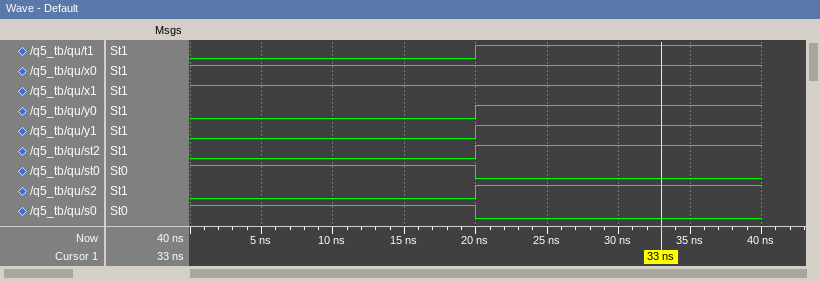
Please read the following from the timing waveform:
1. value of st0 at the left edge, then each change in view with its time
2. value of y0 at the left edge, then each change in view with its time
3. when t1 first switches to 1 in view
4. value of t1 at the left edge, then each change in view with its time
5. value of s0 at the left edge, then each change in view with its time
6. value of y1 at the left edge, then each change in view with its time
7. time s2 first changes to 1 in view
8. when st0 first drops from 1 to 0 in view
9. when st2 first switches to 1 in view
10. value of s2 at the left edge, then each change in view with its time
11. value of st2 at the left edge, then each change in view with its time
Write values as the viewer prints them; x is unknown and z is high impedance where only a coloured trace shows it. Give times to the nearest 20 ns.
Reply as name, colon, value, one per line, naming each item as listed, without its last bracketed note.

value of st0 at the left edge, then each change in view with its time: 1, 0 at 20 ns
value of y0 at the left edge, then each change in view with its time: 0, 1 at 20 ns
when t1 first switches to 1 in view: 20 ns
value of t1 at the left edge, then each change in view with its time: 0, 1 at 20 ns
value of s0 at the left edge, then each change in view with its time: 1, 0 at 20 ns
value of y1 at the left edge, then each change in view with its time: 0, 1 at 20 ns
time s2 first changes to 1 in view: 20 ns
when st0 first drops from 1 to 0 in view: 20 ns
when st2 first switches to 1 in view: 20 ns
value of s2 at the left edge, then each change in view with its time: 0, 1 at 20 ns
value of st2 at the left edge, then each change in view with its time: 0, 1 at 20 ns
